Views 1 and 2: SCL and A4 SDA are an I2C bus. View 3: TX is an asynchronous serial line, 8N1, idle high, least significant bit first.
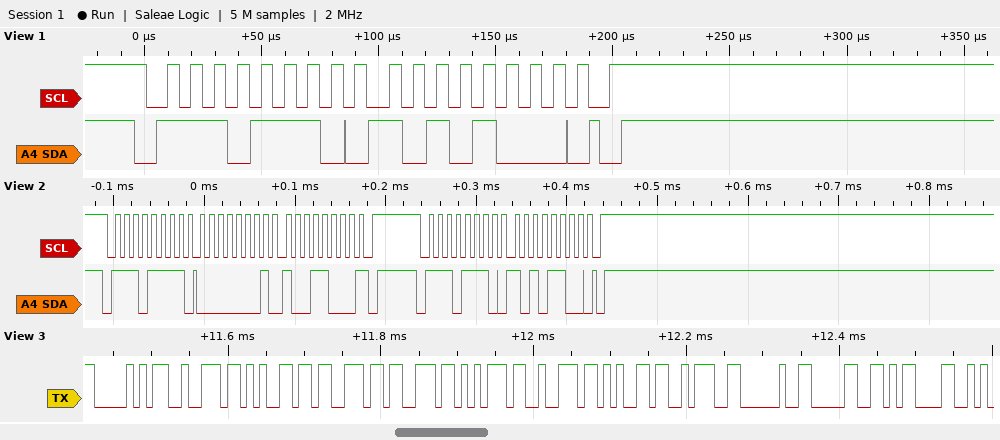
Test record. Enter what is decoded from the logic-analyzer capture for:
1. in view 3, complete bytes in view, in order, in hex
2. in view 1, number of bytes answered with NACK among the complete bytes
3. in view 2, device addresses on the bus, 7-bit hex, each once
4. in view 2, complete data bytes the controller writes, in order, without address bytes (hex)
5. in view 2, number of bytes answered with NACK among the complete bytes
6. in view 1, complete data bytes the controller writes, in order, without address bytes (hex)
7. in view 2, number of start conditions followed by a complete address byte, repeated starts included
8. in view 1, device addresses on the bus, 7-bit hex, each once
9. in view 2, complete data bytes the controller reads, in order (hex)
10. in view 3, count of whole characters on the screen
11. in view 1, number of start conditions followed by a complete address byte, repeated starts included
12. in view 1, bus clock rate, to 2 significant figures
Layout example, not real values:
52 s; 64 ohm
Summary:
50 72 65 73 73 75 72 65 3A 20 30 0D; 0; 0x77; AC; 1; A8; 2; 0x77; 01 98; 12; 1; 100 kHz
